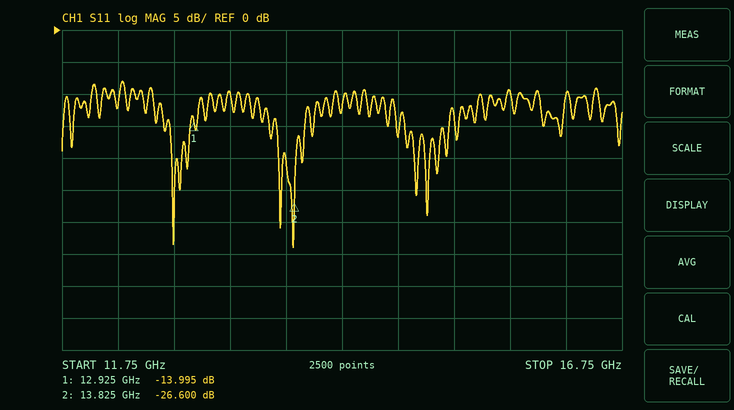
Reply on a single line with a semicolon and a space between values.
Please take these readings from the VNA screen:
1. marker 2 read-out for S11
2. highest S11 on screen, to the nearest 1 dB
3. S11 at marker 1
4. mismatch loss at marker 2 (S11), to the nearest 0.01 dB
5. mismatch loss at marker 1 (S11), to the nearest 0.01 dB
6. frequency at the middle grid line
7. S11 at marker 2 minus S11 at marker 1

-26.600 dB; -8 dB; -13.995 dB; 0.01 dB; 0.18 dB; 14.25 GHz; -12.605 dB
